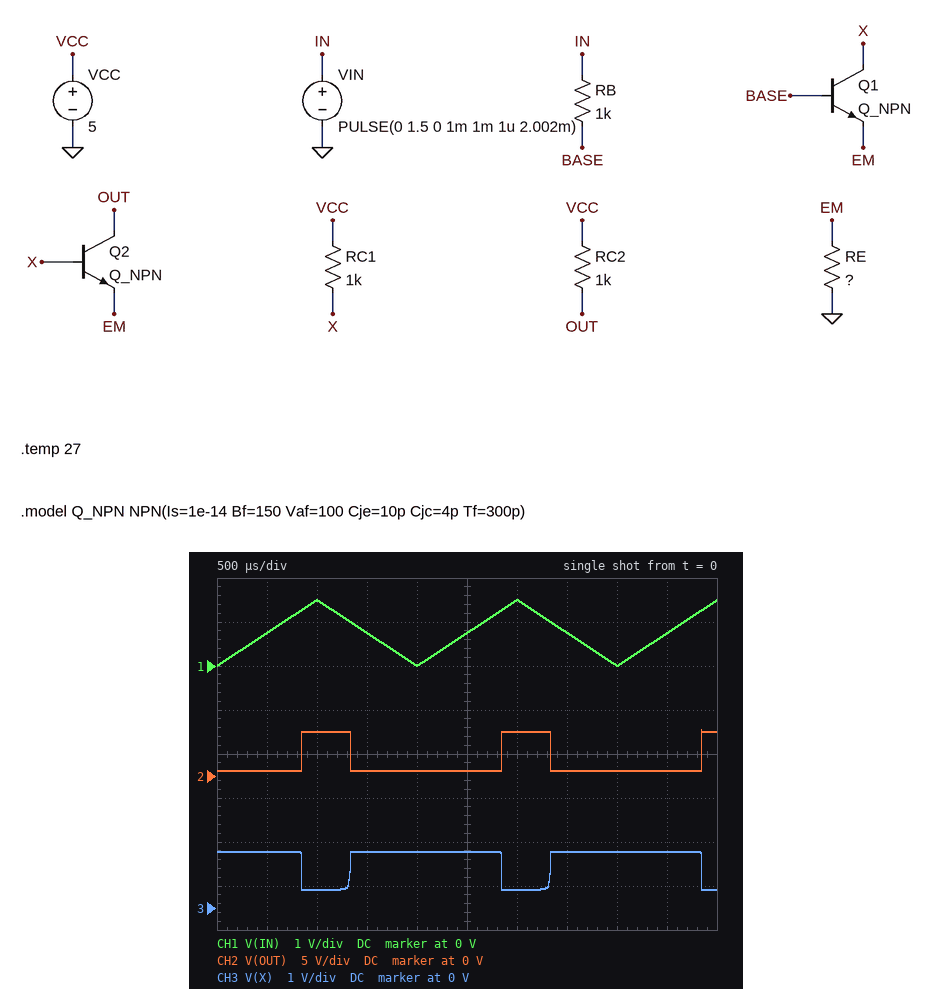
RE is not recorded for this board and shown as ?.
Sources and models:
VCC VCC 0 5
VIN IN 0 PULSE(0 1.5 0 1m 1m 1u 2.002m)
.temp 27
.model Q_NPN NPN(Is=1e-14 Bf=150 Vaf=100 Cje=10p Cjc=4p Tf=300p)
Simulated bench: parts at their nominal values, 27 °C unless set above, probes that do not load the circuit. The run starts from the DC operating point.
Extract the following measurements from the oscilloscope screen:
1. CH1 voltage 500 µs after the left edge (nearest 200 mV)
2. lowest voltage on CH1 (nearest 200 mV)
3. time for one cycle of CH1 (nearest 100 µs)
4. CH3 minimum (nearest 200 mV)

800 mV
0 V
2.0 ms
400 mV
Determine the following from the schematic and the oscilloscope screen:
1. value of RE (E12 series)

68 Ω
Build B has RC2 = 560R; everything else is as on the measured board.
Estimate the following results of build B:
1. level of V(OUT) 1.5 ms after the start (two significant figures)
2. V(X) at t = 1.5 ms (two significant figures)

790 mV
1.5 V
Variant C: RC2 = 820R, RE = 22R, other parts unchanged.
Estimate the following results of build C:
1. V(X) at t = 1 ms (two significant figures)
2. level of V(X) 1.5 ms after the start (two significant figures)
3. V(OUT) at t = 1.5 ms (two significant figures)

180 mV
940 mV
250 mV
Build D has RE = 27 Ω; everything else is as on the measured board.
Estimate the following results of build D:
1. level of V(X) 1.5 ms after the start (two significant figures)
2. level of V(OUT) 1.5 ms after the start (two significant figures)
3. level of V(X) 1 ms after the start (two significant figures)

960 mV
270 mV
210 mV
